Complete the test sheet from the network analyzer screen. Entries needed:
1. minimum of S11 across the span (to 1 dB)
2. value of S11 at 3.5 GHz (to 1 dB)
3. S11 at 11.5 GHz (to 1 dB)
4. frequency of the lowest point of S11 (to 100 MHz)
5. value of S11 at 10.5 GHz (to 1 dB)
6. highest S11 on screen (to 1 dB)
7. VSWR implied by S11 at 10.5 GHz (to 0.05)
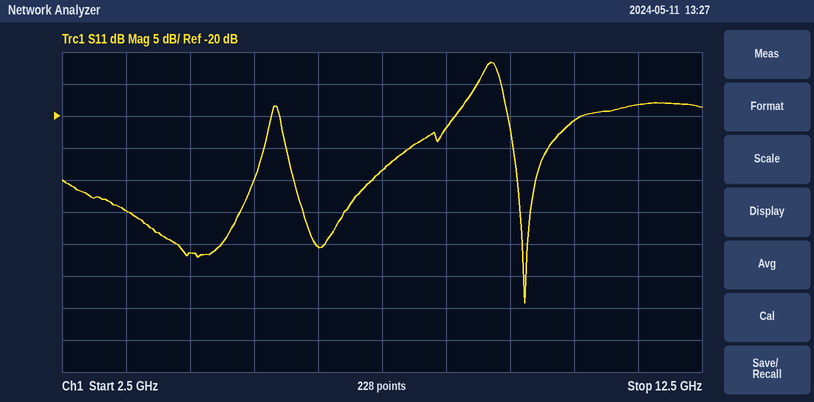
-49 dB
-35 dB
-18 dB
9.7 GHz
-21 dB
-12 dB
1.20
